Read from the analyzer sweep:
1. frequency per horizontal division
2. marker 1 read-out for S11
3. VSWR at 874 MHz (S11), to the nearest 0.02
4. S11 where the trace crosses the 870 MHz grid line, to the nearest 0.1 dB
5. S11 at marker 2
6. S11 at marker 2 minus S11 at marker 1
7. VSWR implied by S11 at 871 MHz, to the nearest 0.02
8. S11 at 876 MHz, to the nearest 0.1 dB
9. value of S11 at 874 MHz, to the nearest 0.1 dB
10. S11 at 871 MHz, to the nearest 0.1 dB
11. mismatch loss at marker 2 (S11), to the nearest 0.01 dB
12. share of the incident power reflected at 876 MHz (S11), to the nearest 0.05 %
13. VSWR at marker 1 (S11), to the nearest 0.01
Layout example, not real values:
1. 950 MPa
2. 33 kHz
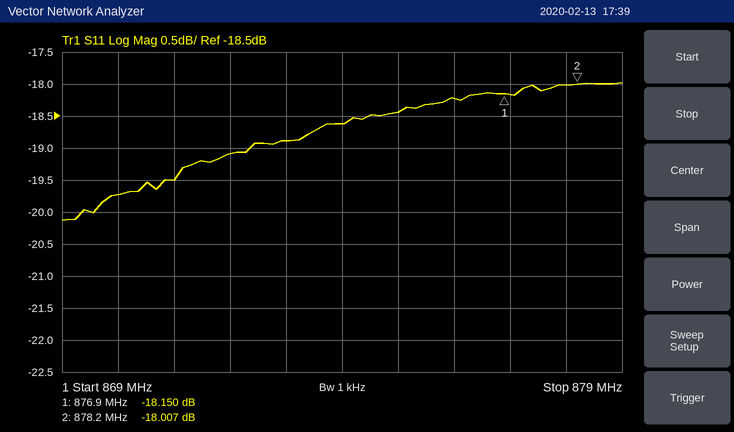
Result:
1. 1 MHz
2. -18.150 dB
3. 1.26
4. -19.7 dB
5. -18.007 dB
6. 0.143 dB
7. 1.24
8. -18.2 dB
9. -18.6 dB
10. -19.5 dB
11. 0.07 dB
12. 1.50 %
13. 1.28
